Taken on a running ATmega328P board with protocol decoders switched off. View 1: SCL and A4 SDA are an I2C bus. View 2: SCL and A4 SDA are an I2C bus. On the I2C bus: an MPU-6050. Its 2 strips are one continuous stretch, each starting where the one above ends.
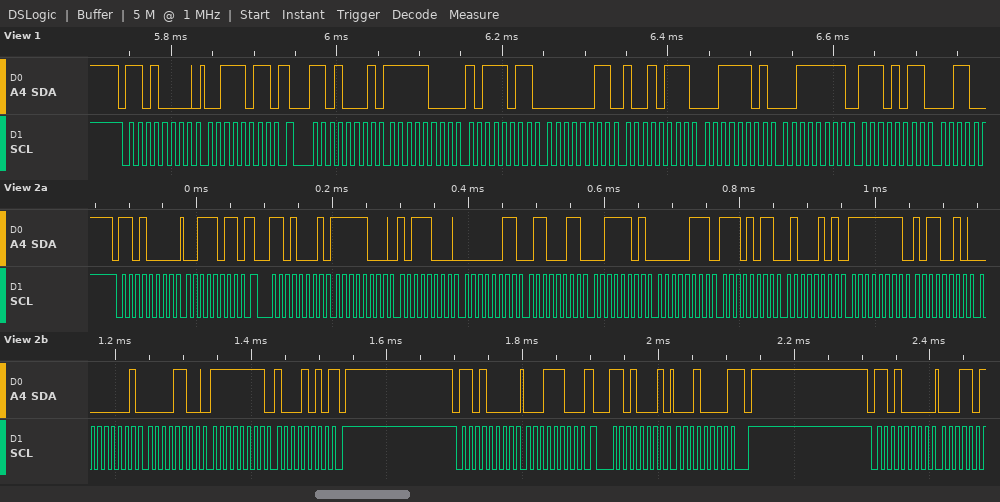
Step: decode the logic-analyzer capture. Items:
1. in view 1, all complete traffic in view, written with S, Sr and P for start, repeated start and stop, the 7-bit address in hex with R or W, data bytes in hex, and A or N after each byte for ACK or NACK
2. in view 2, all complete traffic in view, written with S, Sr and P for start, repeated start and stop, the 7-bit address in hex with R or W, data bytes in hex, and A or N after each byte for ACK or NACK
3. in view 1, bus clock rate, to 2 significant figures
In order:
S 68W A 3B A Sr 68R A F8 A BB A 03 A 97 A 3D A 3F A EB A
S 68W A 3B A Sr 68R A F8 A B8 A 03 A 63 A 3D A 07 A EB A 45 A FF A B2 A 01 A 0C A FF A 8A N P S 68W A 1C A Sr 68R A 10 N P S 68W A
100 kHz
